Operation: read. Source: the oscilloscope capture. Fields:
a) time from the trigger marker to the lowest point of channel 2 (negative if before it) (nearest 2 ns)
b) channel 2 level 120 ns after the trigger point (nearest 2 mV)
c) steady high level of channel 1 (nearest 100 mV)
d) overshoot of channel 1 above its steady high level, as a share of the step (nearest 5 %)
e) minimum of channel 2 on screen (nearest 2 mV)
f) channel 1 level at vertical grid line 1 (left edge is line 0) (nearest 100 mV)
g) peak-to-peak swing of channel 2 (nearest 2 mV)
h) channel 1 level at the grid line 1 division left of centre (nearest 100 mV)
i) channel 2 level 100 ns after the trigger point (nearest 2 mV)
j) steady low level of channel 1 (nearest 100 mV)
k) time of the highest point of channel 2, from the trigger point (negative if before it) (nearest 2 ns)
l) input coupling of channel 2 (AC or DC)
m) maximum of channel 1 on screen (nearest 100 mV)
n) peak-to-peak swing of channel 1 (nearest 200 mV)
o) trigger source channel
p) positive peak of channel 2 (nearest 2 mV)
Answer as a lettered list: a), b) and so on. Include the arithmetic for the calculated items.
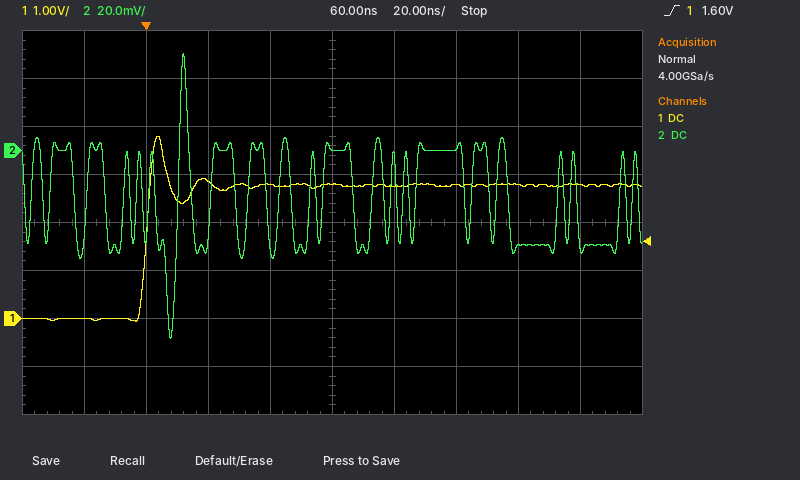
a) +8 ns
b) -40 mV
c) 2.8 V
d) 35 %
e) -78 mV
f) 0.0 V
g) 40 mV − (-78 mV) = 118 mV
h) 2.8 V
i) 2 mV
j) 0.0 V
k) +12 ns
l) DC
m) 3.8 V
n) 3.8 V
o) channel 1
p) 40 mV
